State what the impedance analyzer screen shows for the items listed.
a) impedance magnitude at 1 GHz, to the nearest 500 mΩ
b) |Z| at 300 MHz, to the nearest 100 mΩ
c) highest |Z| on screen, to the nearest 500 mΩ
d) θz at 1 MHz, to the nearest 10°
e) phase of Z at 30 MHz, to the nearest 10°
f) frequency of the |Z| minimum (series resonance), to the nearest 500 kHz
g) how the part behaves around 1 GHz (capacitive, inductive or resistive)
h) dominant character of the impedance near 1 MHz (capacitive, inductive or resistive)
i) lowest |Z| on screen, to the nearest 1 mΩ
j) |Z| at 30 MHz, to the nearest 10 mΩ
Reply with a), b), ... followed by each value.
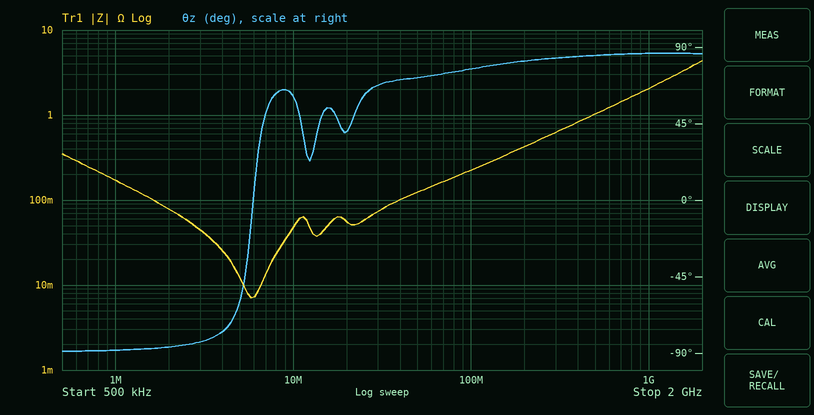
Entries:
a) 2.0 Ω
b) 600 mΩ
c) 4.5 Ω
d) -90°
e) 70°
f) 6.0 MHz
g) inductive
h) capacitive
i) 7 mΩ
j) 70 mΩ
